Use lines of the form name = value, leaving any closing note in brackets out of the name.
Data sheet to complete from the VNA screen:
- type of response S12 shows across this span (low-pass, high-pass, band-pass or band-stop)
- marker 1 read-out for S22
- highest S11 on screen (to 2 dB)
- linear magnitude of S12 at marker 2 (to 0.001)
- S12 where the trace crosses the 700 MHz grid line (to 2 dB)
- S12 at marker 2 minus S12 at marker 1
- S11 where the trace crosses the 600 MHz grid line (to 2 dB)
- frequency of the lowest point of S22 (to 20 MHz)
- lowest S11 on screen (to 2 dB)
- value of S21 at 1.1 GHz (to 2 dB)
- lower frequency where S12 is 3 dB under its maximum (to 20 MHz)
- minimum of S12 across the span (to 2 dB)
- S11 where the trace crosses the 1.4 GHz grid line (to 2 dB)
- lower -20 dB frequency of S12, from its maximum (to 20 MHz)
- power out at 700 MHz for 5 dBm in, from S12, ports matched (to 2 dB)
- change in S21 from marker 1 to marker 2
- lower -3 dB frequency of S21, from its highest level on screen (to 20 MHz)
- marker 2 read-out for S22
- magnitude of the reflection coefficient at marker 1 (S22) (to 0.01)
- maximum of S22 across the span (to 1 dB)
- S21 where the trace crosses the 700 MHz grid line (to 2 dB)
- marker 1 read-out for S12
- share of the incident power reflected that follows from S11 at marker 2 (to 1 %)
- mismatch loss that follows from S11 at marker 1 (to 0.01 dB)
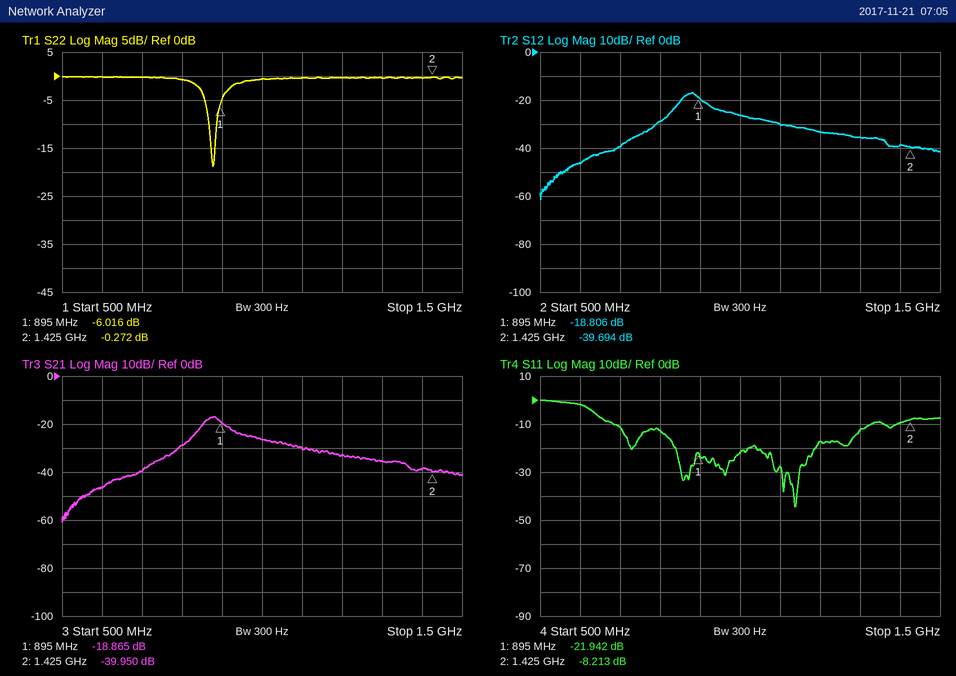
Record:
type of response S12 shows across this span = band-pass
marker 1 read-out for S22 = -6.016 dB
highest S11 on screen = 0 dB
linear magnitude of S12 at marker 2 = 0.010
S12 where the trace crosses the 700 MHz grid line = -40 dB
S12 at marker 2 minus S12 at marker 1 = -20.888 dB
S11 where the trace crosses the 600 MHz grid line = -2 dB
frequency of the lowest point of S22 = 880 MHz
lowest S11 on screen = -44 dB
value of S21 at 1.1 GHz = -30 dB
lower frequency where S12 is 3 dB under its maximum = 860 MHz
minimum of S12 across the span = -62 dB
S11 where the trace crosses the 1.4 GHz grid line = -10 dB
lower -20 dB frequency of S12, from its maximum = 720 MHz
power out at 700 MHz for 5 dBm in, from S12, ports matched = -34 dBm
change in S21 from marker 1 to marker 2 = -21.085 dB
lower -3 dB frequency of S21, from its highest level on screen = 860 MHz
marker 2 read-out for S22 = -0.272 dB
magnitude of the reflection coefficient at marker 1 (S22) = 0.50
maximum of S22 across the span = 0 dB
S21 where the trace crosses the 700 MHz grid line = -40 dB
marker 1 read-out for S12 = -18.806 dB
share of the incident power reflected that follows from S11 at marker 2 = 15 %
mismatch loss that follows from S11 at marker 1 = 0.03 dB
